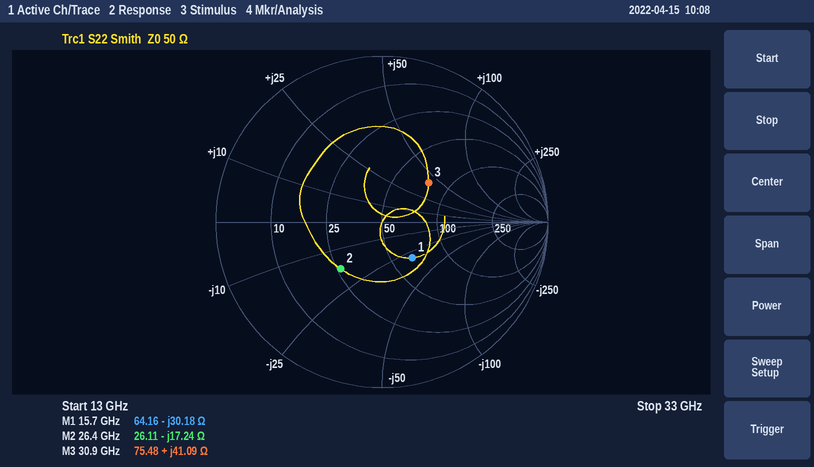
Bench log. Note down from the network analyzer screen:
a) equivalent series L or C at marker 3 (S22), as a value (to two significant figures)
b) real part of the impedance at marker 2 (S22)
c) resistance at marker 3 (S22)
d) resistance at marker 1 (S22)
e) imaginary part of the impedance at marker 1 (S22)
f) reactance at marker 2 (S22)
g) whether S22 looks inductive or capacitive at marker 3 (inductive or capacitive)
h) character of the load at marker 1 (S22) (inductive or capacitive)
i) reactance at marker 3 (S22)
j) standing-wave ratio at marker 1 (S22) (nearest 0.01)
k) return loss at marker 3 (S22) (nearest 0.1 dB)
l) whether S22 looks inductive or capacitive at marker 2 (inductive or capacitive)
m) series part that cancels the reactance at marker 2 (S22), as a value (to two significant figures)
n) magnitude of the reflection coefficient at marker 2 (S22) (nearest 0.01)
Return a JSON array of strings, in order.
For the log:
["210 pH", "26.11 Ω", "75.48 Ω", "64.16 Ω", "-30.18 Ω", "-17.24 Ω", "inductive", "capacitive", "+41.09 Ω", "1.79", "8.7 dB", "capacitive", "100 pH", "0.38"]
